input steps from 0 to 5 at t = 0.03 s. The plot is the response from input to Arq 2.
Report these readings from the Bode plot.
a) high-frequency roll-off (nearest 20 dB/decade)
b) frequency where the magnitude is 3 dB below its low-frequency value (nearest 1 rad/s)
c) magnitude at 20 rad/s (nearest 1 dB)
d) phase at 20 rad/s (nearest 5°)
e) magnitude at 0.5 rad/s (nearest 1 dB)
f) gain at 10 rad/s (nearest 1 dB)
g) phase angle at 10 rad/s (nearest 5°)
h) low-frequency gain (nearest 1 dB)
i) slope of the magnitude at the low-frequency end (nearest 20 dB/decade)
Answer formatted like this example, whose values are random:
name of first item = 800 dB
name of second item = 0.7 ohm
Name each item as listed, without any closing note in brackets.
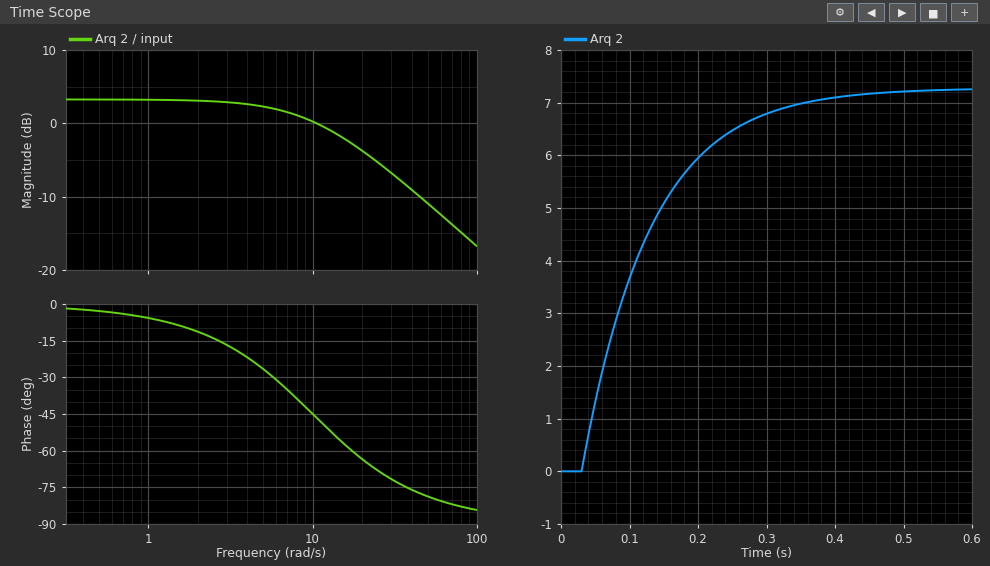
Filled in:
high-frequency roll-off = -20 dB/decade
frequency where the magnitude is 3 dB below its low-frequency value = 10 rad/s
magnitude at 20 rad/s = -4 dB
phase at 20 rad/s = -65°
magnitude at 0.5 rad/s = 3 dB
gain at 10 rad/s = 0 dB
phase angle at 10 rad/s = -45°
low-frequency gain = 3 dB
slope of the magnitude at the low-frequency end = 0 dB/decade
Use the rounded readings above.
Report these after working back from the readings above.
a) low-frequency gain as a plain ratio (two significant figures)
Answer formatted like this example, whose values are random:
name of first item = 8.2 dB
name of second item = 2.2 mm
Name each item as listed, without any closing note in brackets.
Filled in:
low-frequency gain as a plain ratio = 1.4
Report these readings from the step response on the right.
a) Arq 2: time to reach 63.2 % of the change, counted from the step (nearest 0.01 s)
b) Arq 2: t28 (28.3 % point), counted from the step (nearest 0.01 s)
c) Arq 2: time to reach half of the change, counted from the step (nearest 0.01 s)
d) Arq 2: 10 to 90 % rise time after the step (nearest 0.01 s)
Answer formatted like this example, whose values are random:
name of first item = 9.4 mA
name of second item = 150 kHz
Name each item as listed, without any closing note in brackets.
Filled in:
Arq 2: time to reach 63.2 % of the change, counted from the step = 0.10 s
Arq 2: t28 (28.3 % point), counted from the step = 0.03 s
Arq 2: time to reach half of the change, counted from the step = 0.07 s
Arq 2: 10 to 90 % rise time after the step = 0.22 s
